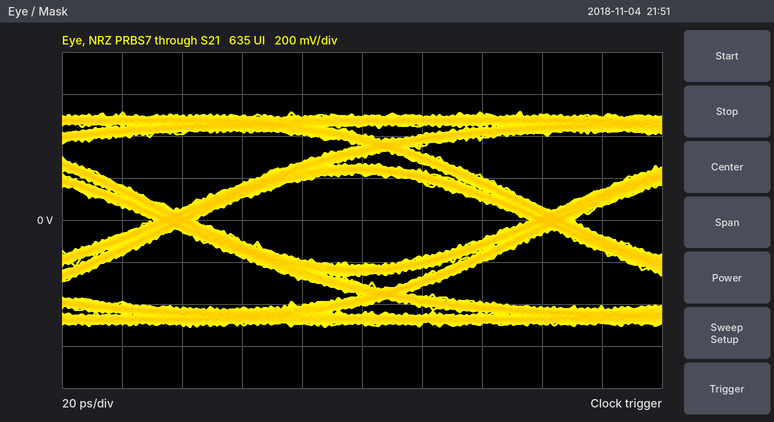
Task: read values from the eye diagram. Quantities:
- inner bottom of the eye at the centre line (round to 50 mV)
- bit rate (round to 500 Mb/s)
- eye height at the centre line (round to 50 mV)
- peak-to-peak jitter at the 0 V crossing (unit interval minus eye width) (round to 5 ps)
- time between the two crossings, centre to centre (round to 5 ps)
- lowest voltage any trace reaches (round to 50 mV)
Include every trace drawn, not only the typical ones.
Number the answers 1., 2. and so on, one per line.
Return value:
1. -200 mV
2. 8.0 Gb/s
3. 450 mV
4. 15 ps
5. 125 ps
6. -500 mV
